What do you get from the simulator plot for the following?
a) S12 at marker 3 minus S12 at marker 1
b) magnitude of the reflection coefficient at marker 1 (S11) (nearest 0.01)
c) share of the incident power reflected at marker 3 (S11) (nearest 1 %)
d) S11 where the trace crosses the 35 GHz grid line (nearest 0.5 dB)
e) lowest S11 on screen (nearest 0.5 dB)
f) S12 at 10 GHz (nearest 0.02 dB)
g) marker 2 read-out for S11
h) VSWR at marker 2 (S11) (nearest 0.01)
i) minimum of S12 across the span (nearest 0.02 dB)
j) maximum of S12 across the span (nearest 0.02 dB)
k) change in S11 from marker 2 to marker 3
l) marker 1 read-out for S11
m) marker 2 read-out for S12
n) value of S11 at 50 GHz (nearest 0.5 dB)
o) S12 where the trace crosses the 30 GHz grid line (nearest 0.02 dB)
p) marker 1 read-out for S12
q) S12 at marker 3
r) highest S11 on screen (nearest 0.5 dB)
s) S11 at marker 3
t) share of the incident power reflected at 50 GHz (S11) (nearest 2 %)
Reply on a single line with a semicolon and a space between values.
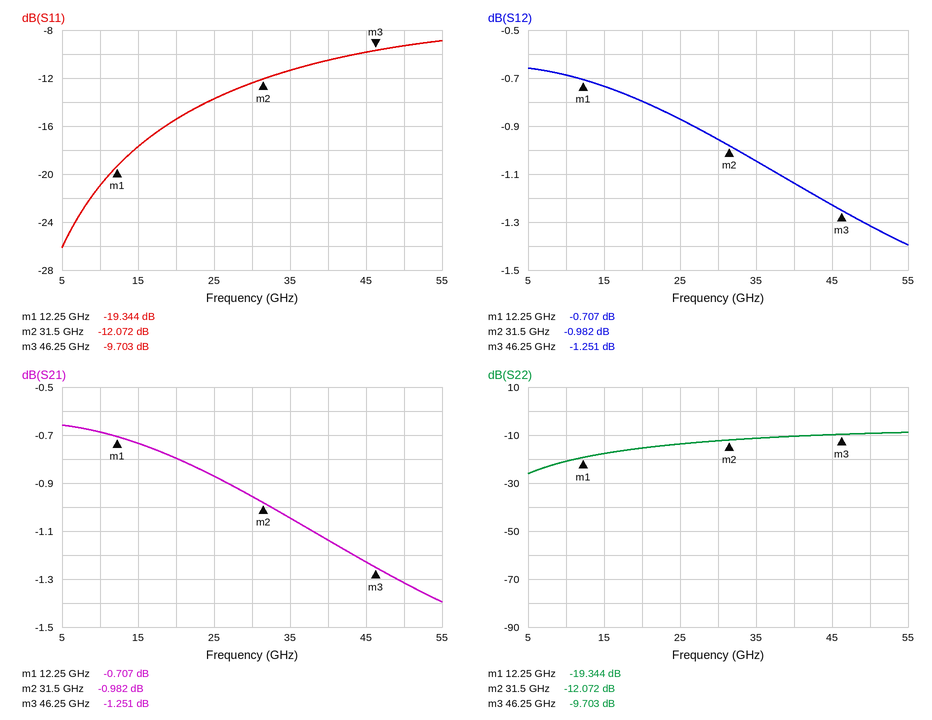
-0.544 dB; 0.11; 11 %; -11.5 dB; -26.0 dB; -0.68 dB; -12.072 dB; 1.66; -1.40 dB; -0.66 dB; 2.369 dB; -19.344 dB; -0.982 dB; -9.5 dB; -0.96 dB; -0.707 dB; -1.251 dB; -9.0 dB; -9.703 dB; 12 %
